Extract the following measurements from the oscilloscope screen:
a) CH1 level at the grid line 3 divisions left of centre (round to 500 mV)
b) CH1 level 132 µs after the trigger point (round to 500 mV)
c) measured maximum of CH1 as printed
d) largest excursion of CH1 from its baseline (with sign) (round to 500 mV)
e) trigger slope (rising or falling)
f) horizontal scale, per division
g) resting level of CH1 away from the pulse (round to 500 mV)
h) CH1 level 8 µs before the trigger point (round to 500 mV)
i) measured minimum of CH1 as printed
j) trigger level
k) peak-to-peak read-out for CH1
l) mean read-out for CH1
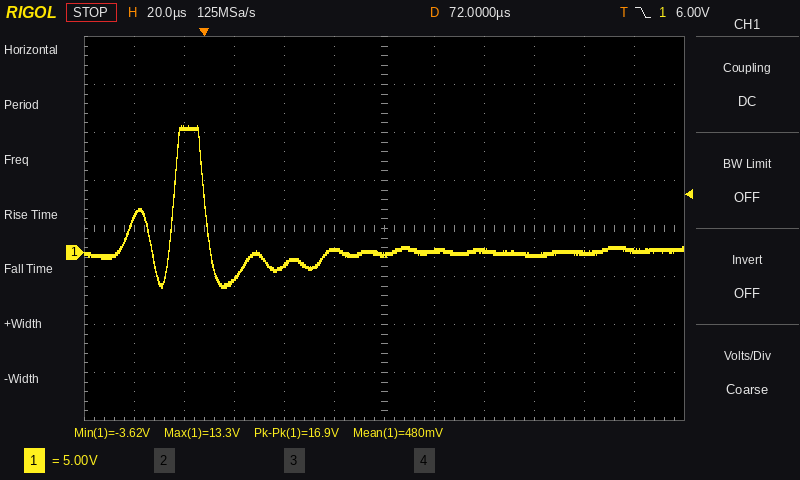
-3.0 V
-500 mV
13.3 V
+13.0 V
falling
20 µs
0.0 V
13.0 V
-3.62 V
6.00 V
16.9 V
480 mV
